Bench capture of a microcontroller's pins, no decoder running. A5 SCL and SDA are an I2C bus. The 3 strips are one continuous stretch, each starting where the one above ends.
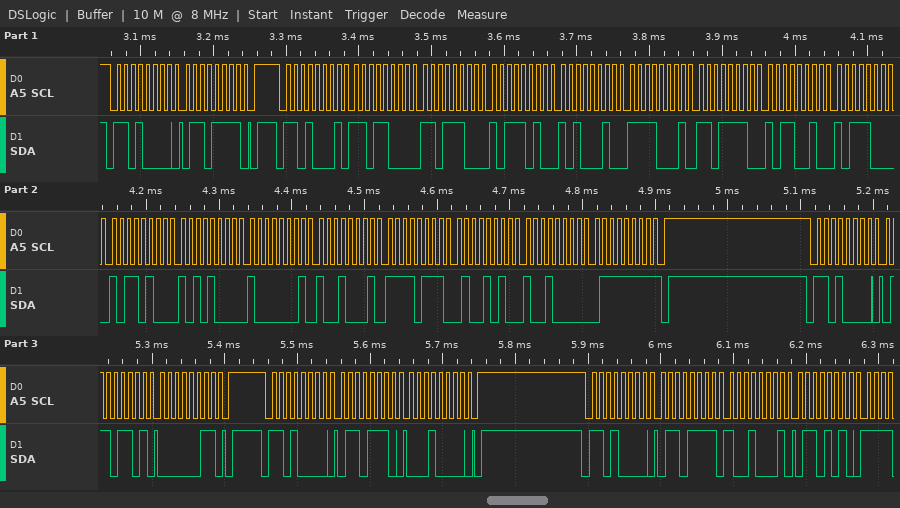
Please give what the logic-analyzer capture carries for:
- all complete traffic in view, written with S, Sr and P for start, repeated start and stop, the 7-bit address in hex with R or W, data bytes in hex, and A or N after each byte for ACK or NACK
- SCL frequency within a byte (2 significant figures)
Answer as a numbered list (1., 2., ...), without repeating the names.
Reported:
1. S 68W A 6F A P S 68R A D8 A DC A BA A A2 A F1 A DE A B2 A B8 A B4 A A8 A 81 A 91 A F7 A 4A A 90 A 7F N P S 68W A 6D A 03 A P S 68W A 6E A 10 A P S 68W A 6F A 91 A 6A A
2. 100 kHz
